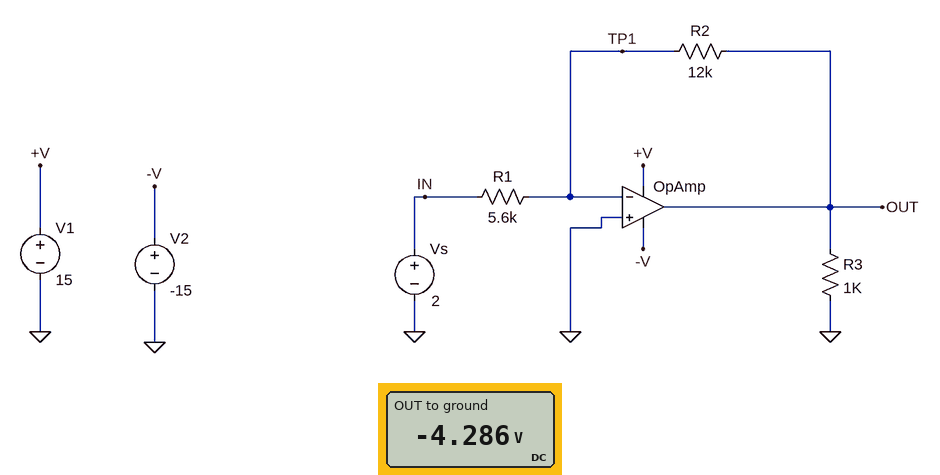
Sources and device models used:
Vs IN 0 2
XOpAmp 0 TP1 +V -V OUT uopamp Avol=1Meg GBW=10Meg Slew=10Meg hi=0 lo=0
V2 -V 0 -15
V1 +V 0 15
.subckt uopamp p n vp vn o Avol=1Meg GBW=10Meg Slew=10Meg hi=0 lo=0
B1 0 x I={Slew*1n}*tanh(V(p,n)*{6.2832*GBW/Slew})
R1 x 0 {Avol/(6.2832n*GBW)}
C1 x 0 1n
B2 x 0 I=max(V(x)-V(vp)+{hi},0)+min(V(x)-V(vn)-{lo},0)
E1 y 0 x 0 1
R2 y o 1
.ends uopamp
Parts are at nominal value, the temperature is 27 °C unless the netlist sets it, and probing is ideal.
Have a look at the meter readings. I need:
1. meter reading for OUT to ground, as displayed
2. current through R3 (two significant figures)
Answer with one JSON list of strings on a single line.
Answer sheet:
["-4.286 V", "4.3 mA"]
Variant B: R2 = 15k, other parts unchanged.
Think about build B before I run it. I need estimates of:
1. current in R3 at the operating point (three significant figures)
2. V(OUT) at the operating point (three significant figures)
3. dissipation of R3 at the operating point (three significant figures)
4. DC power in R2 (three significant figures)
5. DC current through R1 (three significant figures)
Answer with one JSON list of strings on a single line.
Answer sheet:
["5.36 mA", "-5.36 V", "28.7 mW", "1.91 mW", "357 µA"]
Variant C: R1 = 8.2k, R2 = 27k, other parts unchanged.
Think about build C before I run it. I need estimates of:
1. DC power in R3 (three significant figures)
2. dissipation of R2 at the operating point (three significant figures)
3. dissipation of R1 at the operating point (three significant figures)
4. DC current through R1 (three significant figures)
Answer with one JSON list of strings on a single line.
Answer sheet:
["43.4 mW", "1.61 mW", "488 µW", "244 µA"]
